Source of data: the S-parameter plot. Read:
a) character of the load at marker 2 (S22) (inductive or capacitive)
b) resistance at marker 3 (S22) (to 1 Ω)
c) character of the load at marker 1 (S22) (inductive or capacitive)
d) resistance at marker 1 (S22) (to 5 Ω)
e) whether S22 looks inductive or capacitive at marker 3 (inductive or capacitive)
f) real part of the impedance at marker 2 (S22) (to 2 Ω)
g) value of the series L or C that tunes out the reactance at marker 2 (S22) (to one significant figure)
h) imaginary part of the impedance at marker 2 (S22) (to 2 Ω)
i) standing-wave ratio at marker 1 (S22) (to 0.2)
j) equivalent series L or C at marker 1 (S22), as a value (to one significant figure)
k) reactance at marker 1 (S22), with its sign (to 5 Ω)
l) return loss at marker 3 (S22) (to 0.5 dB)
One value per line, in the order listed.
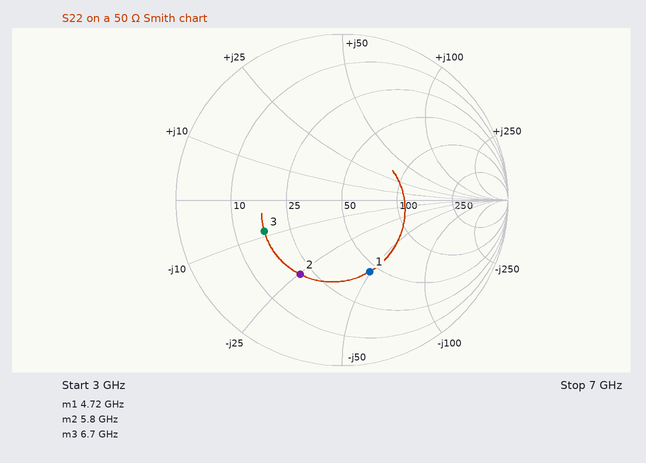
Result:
capacitive
17 Ω
capacitive
45 Ω
capacitive
20 Ω
700 pH
-26 Ω
2.8
700 fF
-50 Ω
6.0 dB
